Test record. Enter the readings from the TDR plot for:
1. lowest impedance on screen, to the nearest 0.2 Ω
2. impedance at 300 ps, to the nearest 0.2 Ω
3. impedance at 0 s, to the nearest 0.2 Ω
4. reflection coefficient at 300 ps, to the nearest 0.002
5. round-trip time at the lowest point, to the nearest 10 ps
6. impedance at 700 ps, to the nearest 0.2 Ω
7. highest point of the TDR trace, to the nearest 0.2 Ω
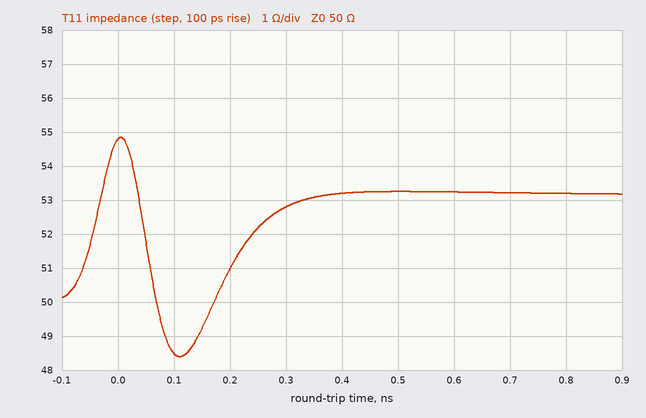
48.4 Ω
52.8 Ω
54.8 Ω
+0.028
110 ps
53.2 Ω
54.8 Ω
